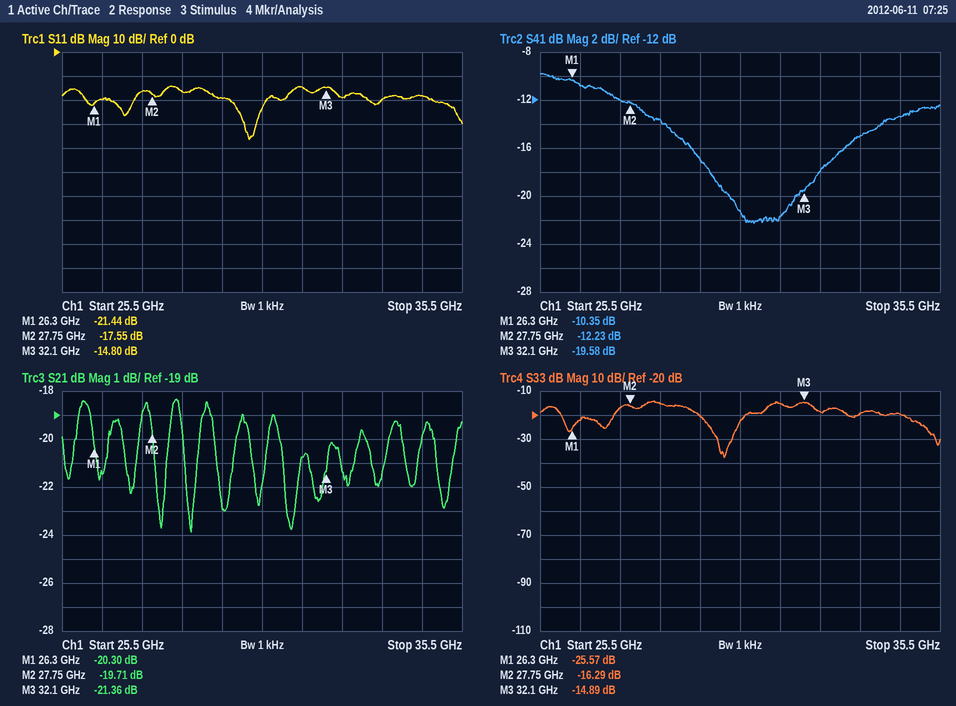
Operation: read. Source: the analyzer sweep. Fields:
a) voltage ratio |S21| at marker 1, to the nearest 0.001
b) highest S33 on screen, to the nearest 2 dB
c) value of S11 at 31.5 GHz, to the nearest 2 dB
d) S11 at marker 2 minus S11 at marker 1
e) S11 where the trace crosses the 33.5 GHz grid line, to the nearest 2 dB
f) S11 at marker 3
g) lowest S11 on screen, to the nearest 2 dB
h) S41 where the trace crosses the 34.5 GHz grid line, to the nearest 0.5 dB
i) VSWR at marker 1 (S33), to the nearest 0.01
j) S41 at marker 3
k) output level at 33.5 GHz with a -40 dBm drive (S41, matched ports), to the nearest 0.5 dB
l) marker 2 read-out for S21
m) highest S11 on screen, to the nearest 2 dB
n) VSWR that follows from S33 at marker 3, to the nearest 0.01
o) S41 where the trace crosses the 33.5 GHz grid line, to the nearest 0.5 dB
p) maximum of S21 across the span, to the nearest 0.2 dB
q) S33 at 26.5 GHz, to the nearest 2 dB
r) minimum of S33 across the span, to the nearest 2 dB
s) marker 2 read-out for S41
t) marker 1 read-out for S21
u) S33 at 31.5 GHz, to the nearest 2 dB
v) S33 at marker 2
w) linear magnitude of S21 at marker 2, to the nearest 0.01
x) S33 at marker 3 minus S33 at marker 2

0.097
-14 dB
-14 dB
3.89 dB
-20 dB
-14.80 dB
-36 dB
-13.5 dB
1.11
-19.58 dB
-55.0 dBm
-19.71 dB
-14 dB
1.44
-15.0 dB
-18.4 dB
-22 dB
-38 dB
-12.23 dB
-20.30 dB
-16 dB
-16.29 dB
0.10
1.40 dB
